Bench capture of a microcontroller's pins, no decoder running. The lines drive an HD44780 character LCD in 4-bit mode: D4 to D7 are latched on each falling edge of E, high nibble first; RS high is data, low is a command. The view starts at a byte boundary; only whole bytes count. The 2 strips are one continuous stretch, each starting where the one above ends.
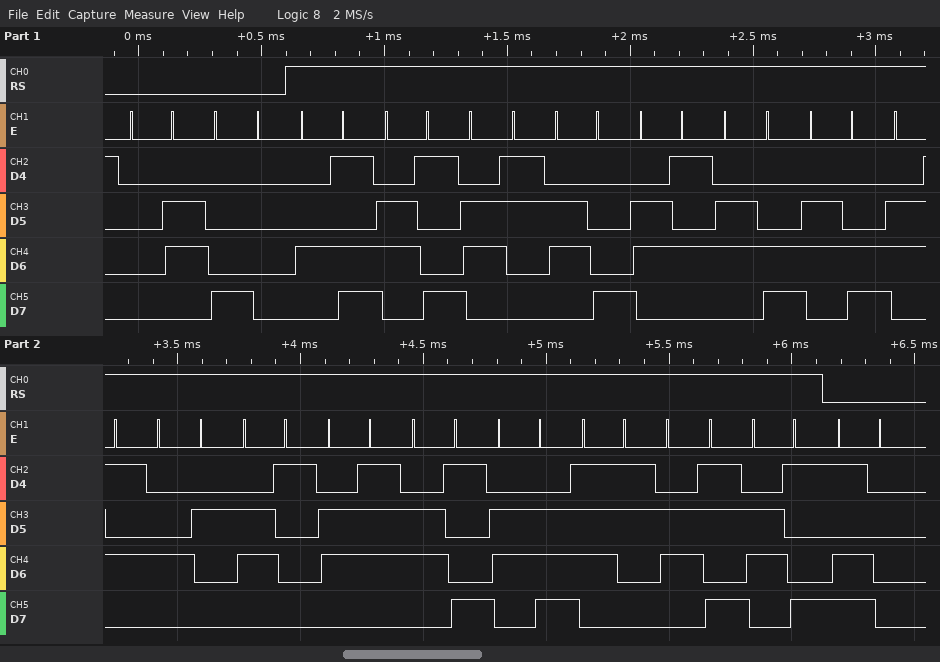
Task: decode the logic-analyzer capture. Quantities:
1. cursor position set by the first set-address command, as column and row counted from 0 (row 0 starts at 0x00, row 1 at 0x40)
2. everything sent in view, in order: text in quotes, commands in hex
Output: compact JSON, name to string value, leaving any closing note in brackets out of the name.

{"cursor position set by the first set-address command, as column and row counted from 0": "column 0, row 0", "everything sent in view, in order: text in quotes, commands in hex": "0x06 0x80 \"MichelleBaginski\" 0xD0"}
